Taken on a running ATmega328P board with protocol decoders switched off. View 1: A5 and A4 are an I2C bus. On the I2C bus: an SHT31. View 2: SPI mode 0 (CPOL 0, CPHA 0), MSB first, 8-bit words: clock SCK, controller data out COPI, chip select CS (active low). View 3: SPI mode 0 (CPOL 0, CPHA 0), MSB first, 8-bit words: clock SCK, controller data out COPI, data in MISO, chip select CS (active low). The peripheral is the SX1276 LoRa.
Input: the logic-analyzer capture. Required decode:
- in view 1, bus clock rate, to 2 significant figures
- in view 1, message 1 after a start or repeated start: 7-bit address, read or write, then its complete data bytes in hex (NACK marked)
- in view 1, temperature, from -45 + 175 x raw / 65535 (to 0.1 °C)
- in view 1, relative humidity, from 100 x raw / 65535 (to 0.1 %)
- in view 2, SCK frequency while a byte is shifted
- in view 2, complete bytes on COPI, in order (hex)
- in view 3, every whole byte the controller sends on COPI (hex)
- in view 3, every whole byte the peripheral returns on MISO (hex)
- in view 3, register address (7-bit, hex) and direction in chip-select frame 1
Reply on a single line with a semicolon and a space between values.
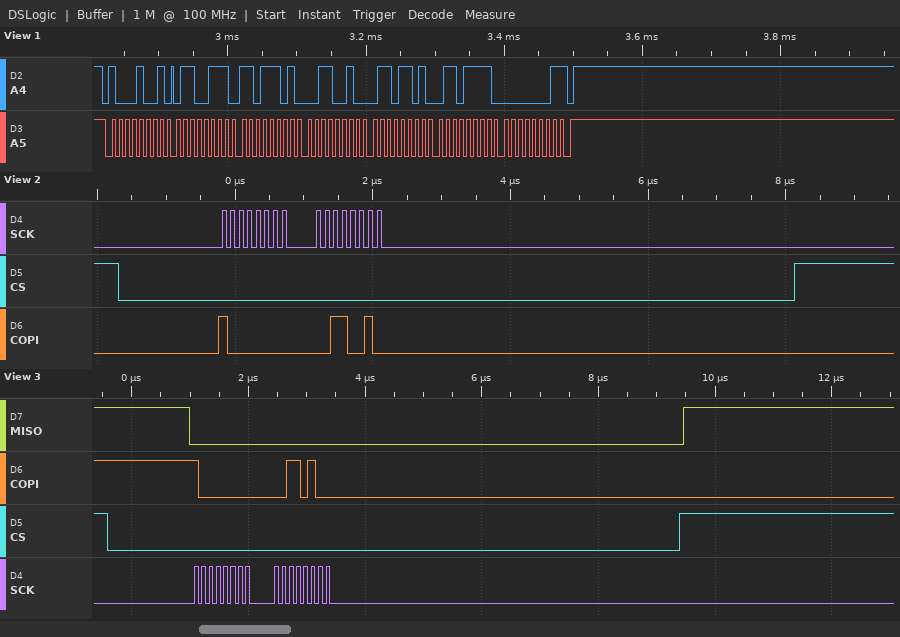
100 kHz; 0x44 read: 67 DD 32 6D 6F 01 NACK; 26.0 °C; 42.7 %; 8 MHz; 80 32; 80 34; 00 00; 0x00 write
